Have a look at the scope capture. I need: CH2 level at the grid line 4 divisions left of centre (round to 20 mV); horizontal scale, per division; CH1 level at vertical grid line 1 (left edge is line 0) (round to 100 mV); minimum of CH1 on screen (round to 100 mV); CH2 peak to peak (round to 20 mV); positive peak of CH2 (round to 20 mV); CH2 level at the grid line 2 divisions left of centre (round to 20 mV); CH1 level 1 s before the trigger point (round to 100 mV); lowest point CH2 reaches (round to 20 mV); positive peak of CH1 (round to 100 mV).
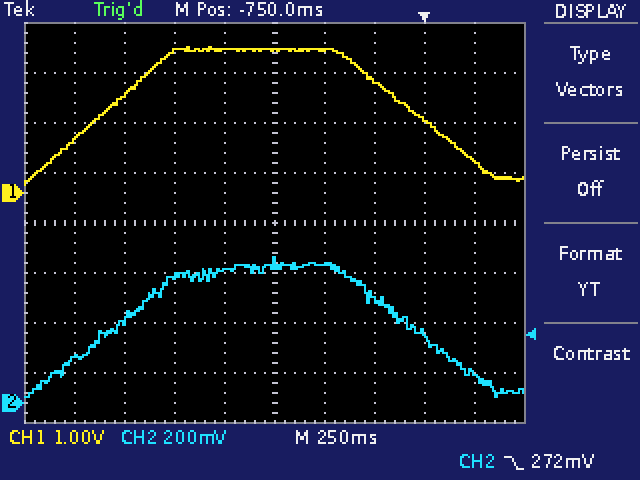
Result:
180 mV
250 ms
1.1 V
200 mV
560 mV
580 mV
500 mV
2.9 V
20 mV
2.9 V
